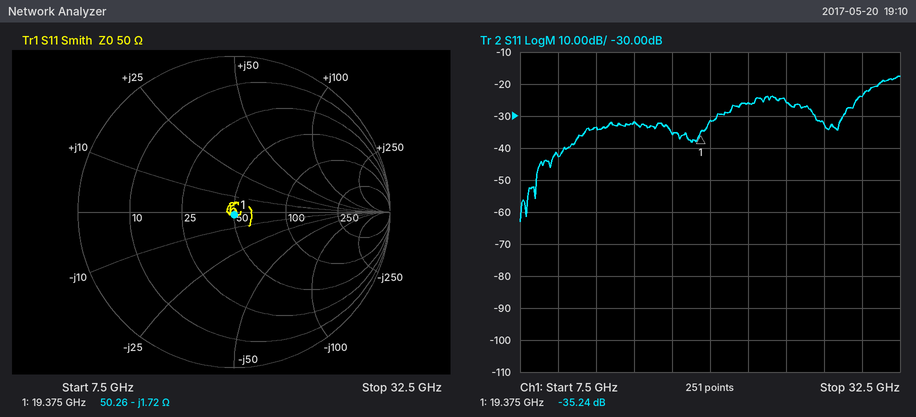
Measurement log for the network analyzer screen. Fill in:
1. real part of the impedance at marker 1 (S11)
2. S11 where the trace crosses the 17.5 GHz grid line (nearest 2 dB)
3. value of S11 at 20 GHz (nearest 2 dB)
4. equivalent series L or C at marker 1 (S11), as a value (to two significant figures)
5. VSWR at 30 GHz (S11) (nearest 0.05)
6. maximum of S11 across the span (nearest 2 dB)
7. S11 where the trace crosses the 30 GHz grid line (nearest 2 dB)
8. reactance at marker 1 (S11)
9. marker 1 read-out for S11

50.26 Ω
-36 dB
-32 dB
4.8 pF
1.15
-18 dB
-24 dB
-1.72 Ω
-35.24 dB
